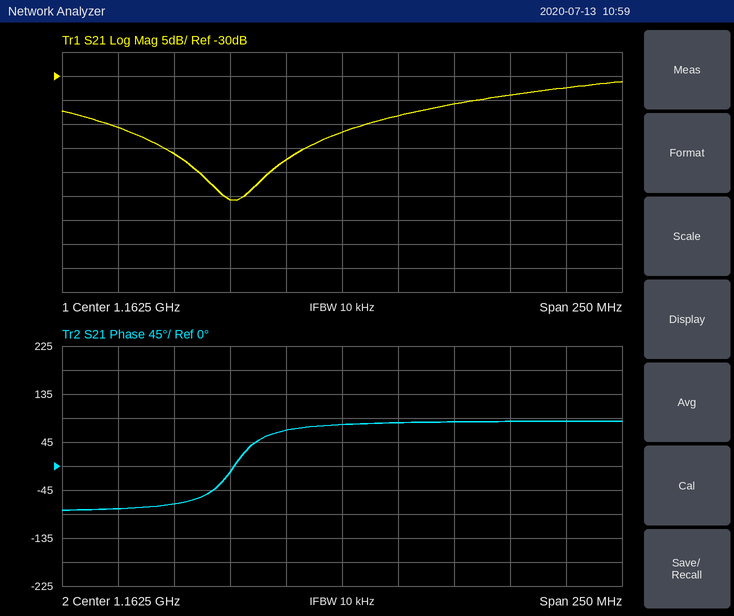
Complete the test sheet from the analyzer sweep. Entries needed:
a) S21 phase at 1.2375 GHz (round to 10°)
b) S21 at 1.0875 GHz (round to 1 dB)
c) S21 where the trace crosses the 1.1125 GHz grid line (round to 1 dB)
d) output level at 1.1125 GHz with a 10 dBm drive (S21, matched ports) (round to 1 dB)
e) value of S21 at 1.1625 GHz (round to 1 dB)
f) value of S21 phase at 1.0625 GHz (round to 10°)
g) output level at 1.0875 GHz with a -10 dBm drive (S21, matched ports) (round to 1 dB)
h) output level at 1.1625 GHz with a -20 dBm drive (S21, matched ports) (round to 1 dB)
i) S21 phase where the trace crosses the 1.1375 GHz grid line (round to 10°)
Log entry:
80°
-46 dB
-56 dB
-46 dBm
-42 dB
-80°
-56 dBm
-62 dBm
70°
